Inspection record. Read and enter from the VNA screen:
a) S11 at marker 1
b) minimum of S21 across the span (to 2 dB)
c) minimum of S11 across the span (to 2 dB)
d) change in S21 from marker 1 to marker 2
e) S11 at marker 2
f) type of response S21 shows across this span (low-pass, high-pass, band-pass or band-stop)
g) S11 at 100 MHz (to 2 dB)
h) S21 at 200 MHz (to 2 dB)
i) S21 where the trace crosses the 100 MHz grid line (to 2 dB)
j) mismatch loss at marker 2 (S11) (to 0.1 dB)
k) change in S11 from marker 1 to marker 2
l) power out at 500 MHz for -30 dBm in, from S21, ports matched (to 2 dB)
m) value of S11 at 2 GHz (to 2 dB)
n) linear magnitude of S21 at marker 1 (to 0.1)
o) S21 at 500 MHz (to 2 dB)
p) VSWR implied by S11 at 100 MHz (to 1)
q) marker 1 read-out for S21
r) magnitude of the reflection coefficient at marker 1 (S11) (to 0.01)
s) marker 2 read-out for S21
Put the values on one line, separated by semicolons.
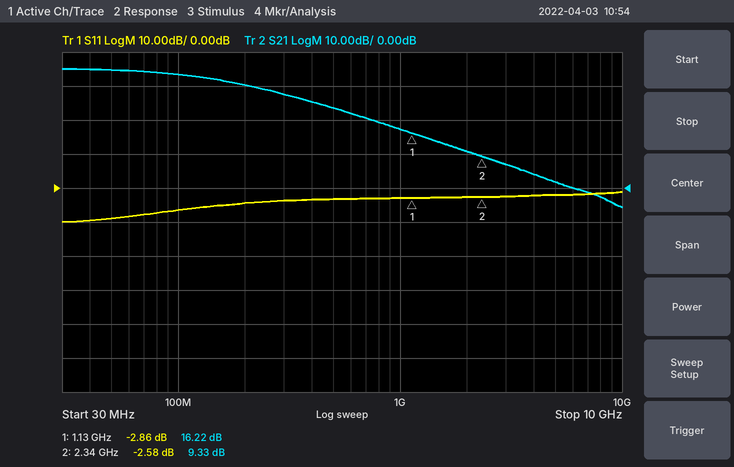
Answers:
-2.86 dB; -6 dB; -10 dB; -6.89 dB; -2.58 dB; low-pass; -6 dB; 30 dB; 34 dB; 3.5 dB; 0.28 dB; -6 dBm; -2 dB; 6.5; 24 dB; 3; 16.22 dB; 0.72; 9.33 dB
